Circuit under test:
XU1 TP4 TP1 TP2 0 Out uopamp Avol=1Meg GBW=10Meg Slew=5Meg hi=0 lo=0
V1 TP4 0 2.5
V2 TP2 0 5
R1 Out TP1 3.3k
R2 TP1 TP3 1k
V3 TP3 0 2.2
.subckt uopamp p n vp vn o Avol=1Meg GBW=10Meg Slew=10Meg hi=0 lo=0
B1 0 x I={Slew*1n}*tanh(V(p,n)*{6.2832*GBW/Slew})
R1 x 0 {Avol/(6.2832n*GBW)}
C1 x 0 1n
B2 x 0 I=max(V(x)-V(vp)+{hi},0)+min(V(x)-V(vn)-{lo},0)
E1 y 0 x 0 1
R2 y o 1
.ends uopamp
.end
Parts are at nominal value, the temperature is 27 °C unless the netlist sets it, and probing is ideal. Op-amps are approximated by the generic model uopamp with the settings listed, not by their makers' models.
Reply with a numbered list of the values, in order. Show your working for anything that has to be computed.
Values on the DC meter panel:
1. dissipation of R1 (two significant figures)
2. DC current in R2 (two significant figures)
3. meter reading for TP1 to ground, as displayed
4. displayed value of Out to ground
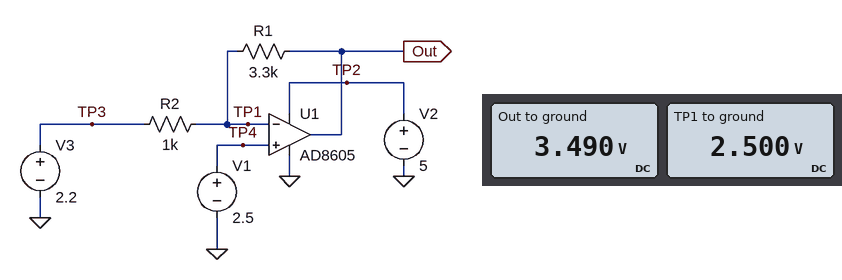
1. (3.49 V - 2.5 V)^2 / 3.3 kΩ = 300 µW
2. (2.5 V - 2.2 V) / 1 kΩ = 300 µA
3. 2.500 V
4. 3.490 V
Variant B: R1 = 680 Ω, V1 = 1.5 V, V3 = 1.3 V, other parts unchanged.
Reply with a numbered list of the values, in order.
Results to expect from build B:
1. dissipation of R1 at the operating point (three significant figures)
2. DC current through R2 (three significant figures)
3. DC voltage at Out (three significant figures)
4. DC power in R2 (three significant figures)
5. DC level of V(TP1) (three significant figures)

1. 27.2 µW
2. 200 µA
3. 1.64 V
4. 40.0 µW
5. 1.50 V
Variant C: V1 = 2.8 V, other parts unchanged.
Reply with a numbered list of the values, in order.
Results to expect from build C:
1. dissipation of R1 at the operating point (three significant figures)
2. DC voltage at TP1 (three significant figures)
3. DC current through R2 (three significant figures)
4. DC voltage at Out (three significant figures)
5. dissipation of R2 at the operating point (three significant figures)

1. 1.19 mW
2. 2.80 V
3. 600 µA
4. 4.78 V
5. 360 µW
